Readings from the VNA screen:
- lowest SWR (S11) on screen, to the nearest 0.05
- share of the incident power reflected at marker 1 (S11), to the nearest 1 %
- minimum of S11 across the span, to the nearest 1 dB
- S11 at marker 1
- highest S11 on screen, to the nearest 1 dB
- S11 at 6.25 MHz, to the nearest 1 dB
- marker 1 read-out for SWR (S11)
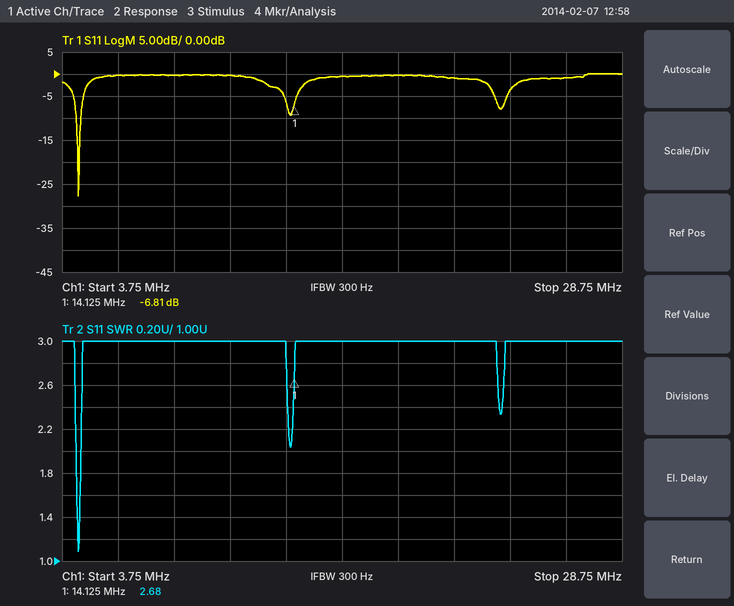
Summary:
1.10
21 %
-28 dB
-6.81 dB
0 dB
0 dB
2.68
